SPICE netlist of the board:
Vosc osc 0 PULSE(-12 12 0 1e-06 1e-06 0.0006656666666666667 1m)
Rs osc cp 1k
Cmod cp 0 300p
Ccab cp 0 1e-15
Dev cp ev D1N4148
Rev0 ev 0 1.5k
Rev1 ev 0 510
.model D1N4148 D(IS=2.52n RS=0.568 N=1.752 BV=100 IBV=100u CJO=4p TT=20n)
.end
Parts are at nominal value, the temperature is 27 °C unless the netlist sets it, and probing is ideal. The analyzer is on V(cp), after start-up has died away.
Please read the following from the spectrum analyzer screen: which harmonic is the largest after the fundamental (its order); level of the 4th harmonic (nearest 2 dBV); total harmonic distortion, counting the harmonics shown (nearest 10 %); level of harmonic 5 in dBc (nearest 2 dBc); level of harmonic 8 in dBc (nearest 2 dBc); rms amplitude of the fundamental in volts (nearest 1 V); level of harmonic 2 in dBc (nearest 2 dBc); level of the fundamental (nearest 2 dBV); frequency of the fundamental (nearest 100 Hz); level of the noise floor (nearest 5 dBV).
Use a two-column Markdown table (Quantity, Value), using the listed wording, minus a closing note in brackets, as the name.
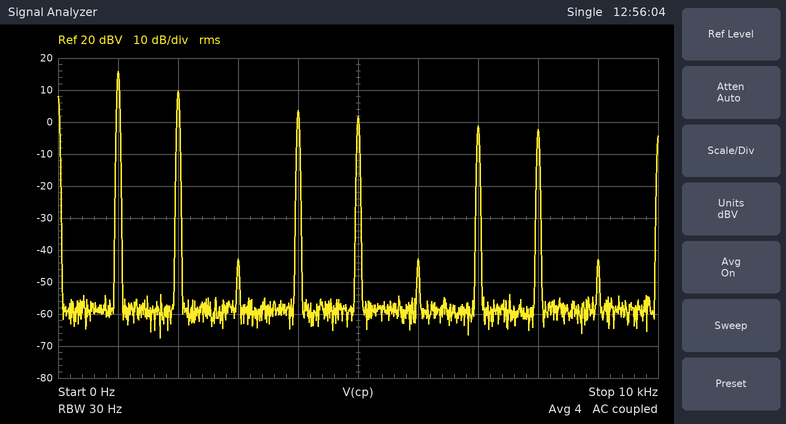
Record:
| Quantity | Value |
|---|---|
| which harmonic is the largest after the fundamental | 2 |
| level of the 4th harmonic | 4 dBV |
| total harmonic distortion, counting the harmonics shown | 60 % |
| level of harmonic 5 in dBc | -14 dBc |
| level of harmonic 8 in dBc | -18 dBc |
| rms amplitude of the fundamental in volts | 6 V |
| level of harmonic 2 in dBc | -6 dBc |
| level of the fundamental | 16 dBV |
| frequency of the fundamental | 1.0 kHz |
| level of the noise floor | -60 dBV |
